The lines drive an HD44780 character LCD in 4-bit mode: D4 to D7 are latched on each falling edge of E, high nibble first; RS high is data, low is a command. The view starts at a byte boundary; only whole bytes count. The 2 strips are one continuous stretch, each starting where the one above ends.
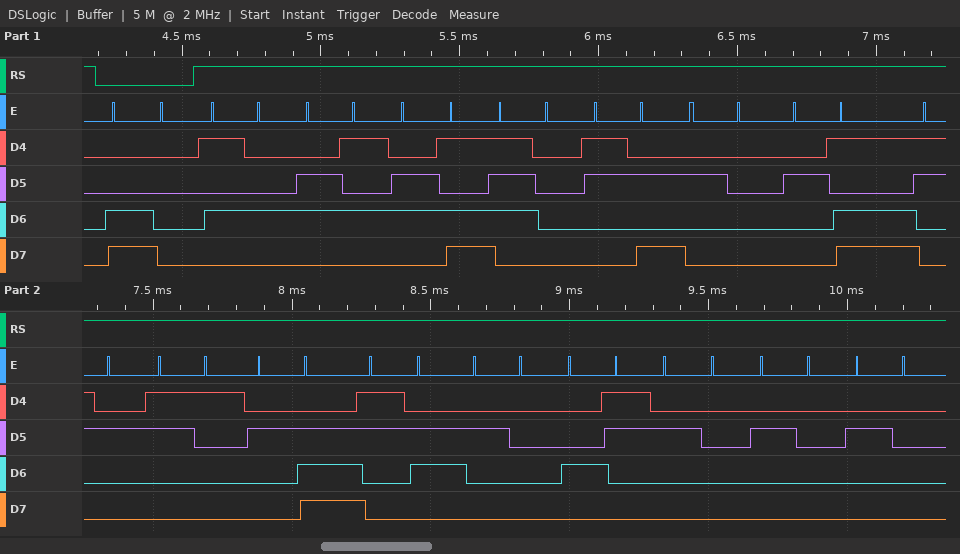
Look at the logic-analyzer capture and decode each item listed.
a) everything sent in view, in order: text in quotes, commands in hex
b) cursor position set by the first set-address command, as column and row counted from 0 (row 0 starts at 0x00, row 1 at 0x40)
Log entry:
0xC0 "Temp: -21.6 C   "
column 0, row 1
